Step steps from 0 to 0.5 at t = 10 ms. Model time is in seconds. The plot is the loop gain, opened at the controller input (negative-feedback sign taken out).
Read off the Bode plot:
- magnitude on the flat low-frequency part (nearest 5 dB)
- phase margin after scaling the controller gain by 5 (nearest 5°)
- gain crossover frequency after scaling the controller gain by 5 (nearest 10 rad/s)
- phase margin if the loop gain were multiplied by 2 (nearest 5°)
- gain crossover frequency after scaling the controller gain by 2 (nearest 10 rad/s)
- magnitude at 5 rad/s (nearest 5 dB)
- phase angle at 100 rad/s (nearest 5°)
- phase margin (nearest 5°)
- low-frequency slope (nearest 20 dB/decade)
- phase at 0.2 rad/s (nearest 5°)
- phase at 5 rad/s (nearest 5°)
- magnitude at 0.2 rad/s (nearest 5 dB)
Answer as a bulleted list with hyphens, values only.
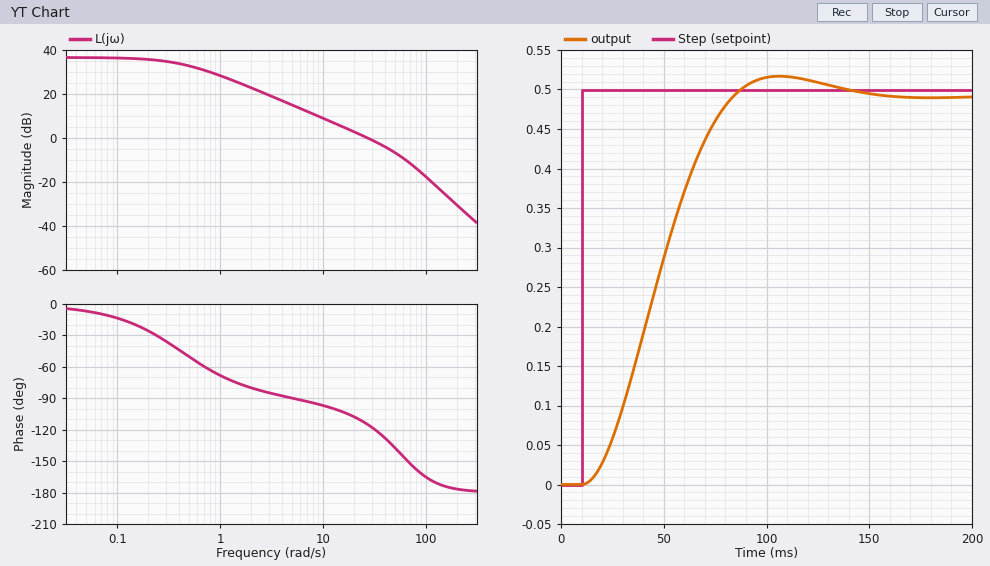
- 35 dB
- 20°
- 80 rad/s
- 45°
- 50 rad/s
- 15 dB
- -165°
- 65°
- 0 dB/decade
- -25°
- -90°
- 35 dB
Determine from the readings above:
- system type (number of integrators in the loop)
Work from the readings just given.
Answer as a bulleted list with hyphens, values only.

- 0
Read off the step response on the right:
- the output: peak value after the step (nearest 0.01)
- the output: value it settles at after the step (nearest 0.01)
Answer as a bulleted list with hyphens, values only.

- 0.52
- 0.49
